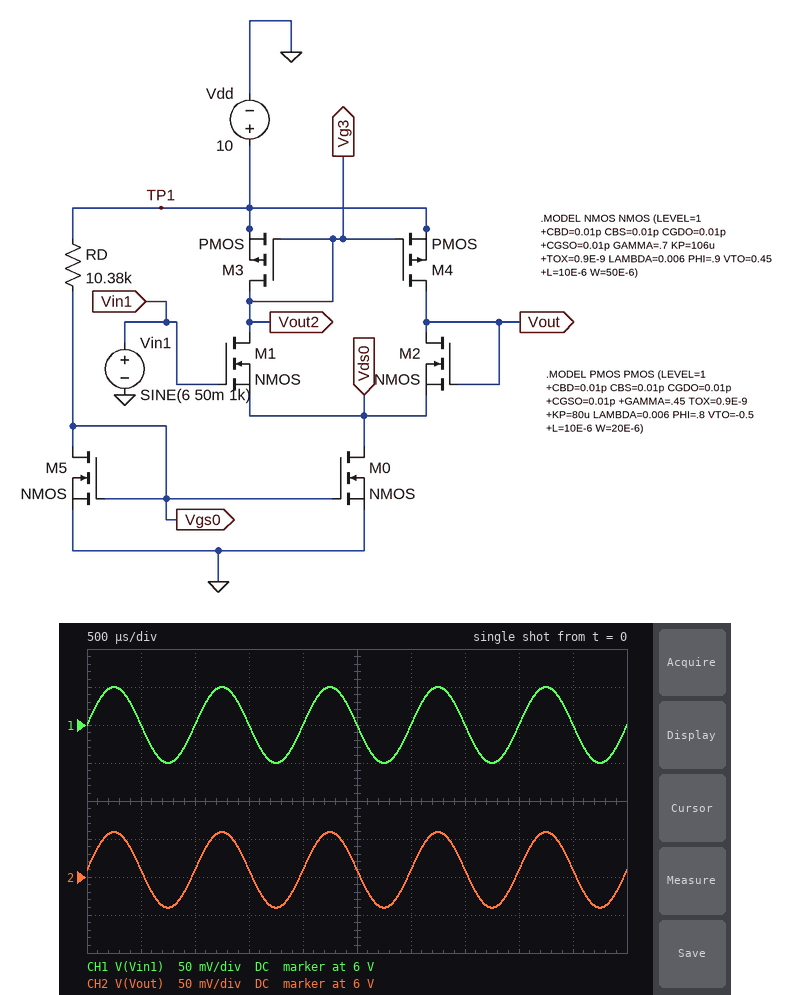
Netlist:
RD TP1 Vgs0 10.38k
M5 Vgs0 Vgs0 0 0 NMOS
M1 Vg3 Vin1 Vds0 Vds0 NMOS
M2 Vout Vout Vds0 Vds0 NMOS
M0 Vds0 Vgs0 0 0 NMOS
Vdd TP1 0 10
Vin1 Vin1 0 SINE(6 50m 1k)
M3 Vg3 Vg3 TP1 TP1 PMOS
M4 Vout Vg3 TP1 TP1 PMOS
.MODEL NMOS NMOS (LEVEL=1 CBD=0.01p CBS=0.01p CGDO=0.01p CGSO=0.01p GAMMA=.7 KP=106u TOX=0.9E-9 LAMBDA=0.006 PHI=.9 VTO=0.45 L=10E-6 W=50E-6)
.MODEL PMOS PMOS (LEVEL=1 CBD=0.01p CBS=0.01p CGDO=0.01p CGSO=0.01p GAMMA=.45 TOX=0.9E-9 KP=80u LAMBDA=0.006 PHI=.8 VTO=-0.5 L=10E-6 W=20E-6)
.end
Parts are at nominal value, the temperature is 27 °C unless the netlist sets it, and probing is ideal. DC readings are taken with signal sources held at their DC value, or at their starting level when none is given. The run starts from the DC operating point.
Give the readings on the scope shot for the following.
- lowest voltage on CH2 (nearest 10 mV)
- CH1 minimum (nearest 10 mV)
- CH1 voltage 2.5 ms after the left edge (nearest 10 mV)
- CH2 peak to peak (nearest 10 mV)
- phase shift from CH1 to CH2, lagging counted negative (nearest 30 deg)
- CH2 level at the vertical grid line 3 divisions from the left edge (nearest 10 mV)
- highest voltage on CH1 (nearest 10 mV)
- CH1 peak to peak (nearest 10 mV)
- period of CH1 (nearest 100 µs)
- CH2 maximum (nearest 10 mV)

5.96 V
5.95 V
6.00 V
100 mV
0 deg
6.01 V
6.05 V
100 mV
1.0 ms
6.06 V
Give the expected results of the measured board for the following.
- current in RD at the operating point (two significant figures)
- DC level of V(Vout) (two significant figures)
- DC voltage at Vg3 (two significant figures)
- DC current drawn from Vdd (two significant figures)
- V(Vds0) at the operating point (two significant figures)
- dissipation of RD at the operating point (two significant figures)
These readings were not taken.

760 µA
6.0 V
7.3 V
1.5 mA
4.4 V
6.0 mW
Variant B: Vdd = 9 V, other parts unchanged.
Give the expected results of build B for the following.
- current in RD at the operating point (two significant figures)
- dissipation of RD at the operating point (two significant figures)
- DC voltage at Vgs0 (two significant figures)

670 µA
4.7 mW
2.0 V
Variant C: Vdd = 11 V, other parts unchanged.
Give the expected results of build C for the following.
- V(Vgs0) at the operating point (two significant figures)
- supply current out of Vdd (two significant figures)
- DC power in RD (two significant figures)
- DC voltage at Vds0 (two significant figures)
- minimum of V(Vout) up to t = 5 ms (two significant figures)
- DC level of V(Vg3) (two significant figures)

2.2 V
1.7 mA
7.4 mW
4.3 V
6.0 V
8.2 V
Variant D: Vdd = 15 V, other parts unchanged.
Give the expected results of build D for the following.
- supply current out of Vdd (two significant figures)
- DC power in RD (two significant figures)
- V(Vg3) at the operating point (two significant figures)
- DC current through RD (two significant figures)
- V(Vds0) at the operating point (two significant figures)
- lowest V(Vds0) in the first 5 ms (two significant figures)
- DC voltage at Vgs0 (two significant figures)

2.4 mA
15 mW
12 V
1.2 mA
4.1 V
4.0 V
2.6 V
